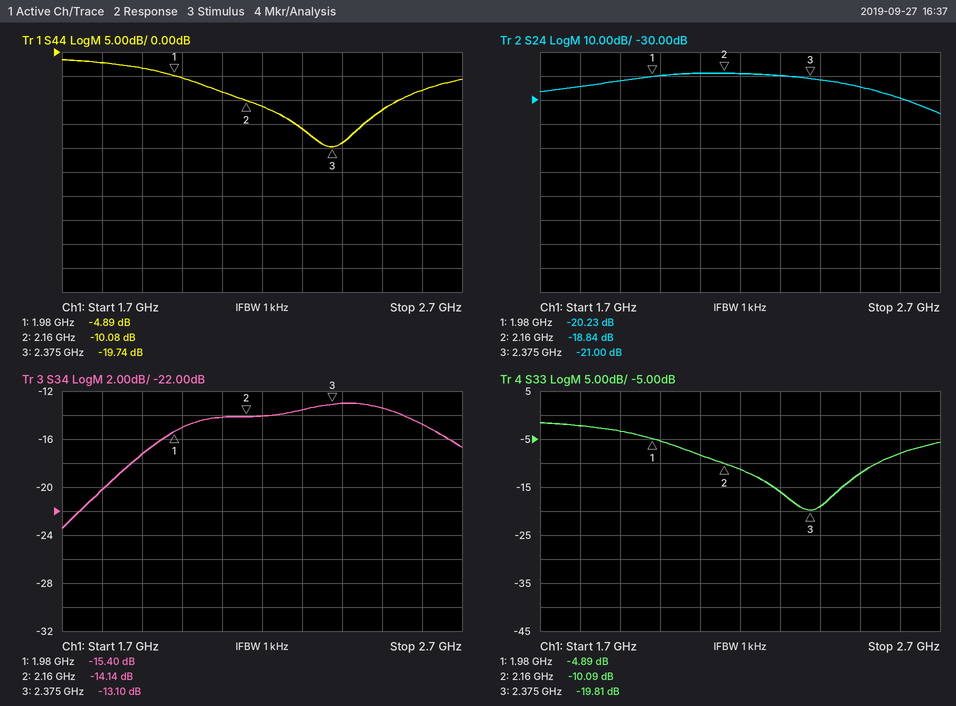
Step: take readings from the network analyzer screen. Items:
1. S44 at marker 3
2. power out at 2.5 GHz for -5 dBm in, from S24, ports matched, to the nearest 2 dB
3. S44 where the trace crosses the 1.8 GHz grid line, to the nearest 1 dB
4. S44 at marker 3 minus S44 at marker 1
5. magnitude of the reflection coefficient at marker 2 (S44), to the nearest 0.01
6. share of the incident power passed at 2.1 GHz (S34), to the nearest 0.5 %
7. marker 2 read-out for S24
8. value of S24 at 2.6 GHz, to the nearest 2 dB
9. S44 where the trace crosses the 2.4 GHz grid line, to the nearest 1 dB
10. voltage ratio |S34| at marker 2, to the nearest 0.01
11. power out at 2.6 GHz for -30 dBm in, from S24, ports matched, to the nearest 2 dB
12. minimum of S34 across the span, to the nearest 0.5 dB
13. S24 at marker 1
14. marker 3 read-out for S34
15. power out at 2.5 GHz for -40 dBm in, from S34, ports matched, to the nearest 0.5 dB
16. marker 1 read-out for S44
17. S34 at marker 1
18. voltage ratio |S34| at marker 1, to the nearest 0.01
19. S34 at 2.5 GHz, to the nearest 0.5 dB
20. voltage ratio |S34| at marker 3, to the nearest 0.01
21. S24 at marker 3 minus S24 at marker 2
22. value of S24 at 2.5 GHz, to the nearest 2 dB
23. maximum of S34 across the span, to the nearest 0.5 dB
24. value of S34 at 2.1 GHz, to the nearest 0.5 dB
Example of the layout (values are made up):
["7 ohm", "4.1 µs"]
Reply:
["-19.74 dB", "-30 dBm", "-2 dB", "-14.85 dB", "0.31", "4.0 %", "-18.84 dB", "-30 dB", "-19 dB", "0.20", "-60 dBm", "-23.5 dB", "-20.23 dB", "-13.10 dB", "-53.5 dBm", "-4.89 dB", "-15.40 dB", "0.17", "-13.5 dB", "0.22", "-2.16 dB", "-24 dB", "-13.0 dB", "-14.0 dB"]
